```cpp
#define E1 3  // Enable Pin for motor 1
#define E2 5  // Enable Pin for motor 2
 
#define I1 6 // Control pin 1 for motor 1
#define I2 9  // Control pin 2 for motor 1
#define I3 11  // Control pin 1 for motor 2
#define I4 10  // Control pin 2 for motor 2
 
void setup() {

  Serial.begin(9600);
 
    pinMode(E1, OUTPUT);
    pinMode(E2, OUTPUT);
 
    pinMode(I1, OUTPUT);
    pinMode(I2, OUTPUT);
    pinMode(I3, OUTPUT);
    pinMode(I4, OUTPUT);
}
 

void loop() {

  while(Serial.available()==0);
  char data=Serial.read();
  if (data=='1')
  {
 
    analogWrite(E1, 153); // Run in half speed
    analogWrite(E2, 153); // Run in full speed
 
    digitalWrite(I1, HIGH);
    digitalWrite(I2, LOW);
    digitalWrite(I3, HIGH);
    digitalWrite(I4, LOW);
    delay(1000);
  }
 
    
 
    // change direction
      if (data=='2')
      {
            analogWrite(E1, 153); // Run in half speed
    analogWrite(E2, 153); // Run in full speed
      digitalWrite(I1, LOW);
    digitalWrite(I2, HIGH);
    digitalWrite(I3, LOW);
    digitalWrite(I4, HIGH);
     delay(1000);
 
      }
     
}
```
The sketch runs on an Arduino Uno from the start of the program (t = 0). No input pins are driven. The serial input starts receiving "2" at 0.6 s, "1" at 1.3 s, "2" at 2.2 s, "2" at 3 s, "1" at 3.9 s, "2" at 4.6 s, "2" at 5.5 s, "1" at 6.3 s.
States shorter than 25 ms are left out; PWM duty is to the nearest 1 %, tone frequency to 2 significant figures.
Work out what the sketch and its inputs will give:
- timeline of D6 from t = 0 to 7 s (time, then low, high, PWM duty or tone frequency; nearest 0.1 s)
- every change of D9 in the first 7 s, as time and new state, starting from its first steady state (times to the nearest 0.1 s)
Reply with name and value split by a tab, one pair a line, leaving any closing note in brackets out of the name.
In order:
timeline of D6 from t = 0 to 7 s	0 s low; 1.6 s high; 2.6 s low; 4.6 s high; 5.6 s low
every change of D9 in the first 7 s, as time and new state, starting from its first steady state	0 s low; 0.6 s high; 1.6 s low; 2.6 s high; 4.6 s low; 5.6 s high
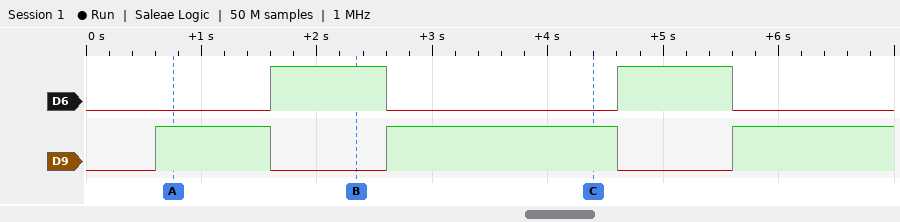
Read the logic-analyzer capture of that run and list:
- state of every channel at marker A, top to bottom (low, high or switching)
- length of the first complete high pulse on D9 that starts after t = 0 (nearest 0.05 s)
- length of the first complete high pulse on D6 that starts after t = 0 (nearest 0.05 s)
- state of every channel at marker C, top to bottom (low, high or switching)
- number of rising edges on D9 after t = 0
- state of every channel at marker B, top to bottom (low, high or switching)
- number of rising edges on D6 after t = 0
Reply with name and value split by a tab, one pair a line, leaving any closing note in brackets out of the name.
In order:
state of every channel at marker A, top to bottom	D6 low, D9 high
length of the first complete high pulse on D9 that starts after t = 0	1.00 s
length of the first complete high pulse on D6 that starts after t = 0	1.00 s
state of every channel at marker C, top to bottom	D6 low, D9 high
number of rising edges on D9 after t = 0	3
state of every channel at marker B, top to bottom	D6 high, D9 low
number of rising edges on D6 after t = 0	2
